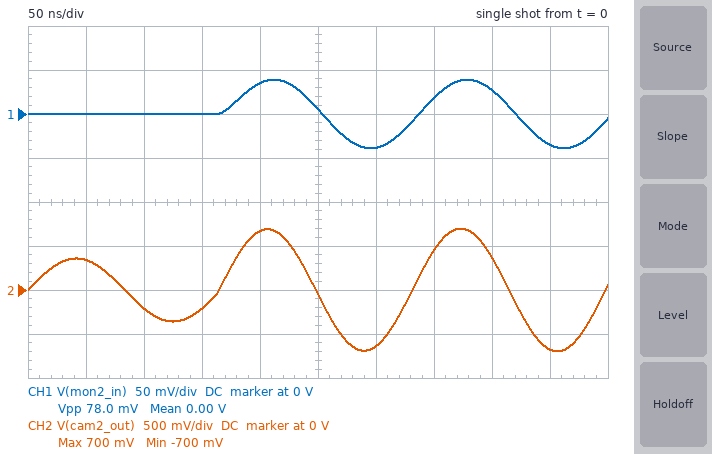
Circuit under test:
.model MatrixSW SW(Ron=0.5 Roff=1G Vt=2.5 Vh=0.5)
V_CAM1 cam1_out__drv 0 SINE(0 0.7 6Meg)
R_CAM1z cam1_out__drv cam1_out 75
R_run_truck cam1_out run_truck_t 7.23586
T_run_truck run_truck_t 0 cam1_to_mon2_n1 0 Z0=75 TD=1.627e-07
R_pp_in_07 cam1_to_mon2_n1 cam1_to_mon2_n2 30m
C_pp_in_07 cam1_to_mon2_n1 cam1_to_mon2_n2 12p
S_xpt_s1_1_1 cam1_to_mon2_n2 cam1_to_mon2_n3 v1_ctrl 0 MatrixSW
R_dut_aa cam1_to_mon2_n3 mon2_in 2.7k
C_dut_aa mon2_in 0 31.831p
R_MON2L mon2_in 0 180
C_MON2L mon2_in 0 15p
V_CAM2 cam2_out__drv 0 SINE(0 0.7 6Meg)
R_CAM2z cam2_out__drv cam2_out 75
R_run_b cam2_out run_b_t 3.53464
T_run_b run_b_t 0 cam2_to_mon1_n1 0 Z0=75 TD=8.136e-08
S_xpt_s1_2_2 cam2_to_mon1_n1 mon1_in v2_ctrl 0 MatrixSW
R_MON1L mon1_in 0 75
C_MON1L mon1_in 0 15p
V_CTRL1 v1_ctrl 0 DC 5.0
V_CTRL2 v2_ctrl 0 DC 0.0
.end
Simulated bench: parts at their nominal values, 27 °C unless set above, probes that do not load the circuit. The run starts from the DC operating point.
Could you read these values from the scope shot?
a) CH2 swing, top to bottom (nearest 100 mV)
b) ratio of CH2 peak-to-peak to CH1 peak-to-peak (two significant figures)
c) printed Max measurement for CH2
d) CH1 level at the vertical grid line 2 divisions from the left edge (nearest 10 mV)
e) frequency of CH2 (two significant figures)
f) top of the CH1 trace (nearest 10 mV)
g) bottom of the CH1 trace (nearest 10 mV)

1.4 V
18
700 mV
0 V
6.0 MHz
40 mV
-40 mV
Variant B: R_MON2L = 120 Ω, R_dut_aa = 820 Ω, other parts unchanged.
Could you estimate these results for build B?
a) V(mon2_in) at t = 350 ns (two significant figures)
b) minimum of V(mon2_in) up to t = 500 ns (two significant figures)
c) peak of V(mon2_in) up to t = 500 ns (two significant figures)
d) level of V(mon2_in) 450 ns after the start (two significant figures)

43 mV
-78 mV
78 mV
-73 mV
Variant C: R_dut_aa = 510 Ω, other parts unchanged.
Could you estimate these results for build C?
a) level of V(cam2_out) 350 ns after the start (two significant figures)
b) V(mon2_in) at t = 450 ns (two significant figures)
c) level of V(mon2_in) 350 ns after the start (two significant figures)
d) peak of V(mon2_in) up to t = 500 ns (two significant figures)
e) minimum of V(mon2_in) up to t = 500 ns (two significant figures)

450 mV
-140 mV
78 mV
150 mV
-150 mV
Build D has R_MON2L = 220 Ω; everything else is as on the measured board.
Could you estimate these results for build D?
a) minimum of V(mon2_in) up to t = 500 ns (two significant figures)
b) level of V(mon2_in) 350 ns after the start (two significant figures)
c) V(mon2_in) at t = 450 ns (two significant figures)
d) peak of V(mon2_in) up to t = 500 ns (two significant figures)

-46 mV
19 mV
-40 mV
46 mV
